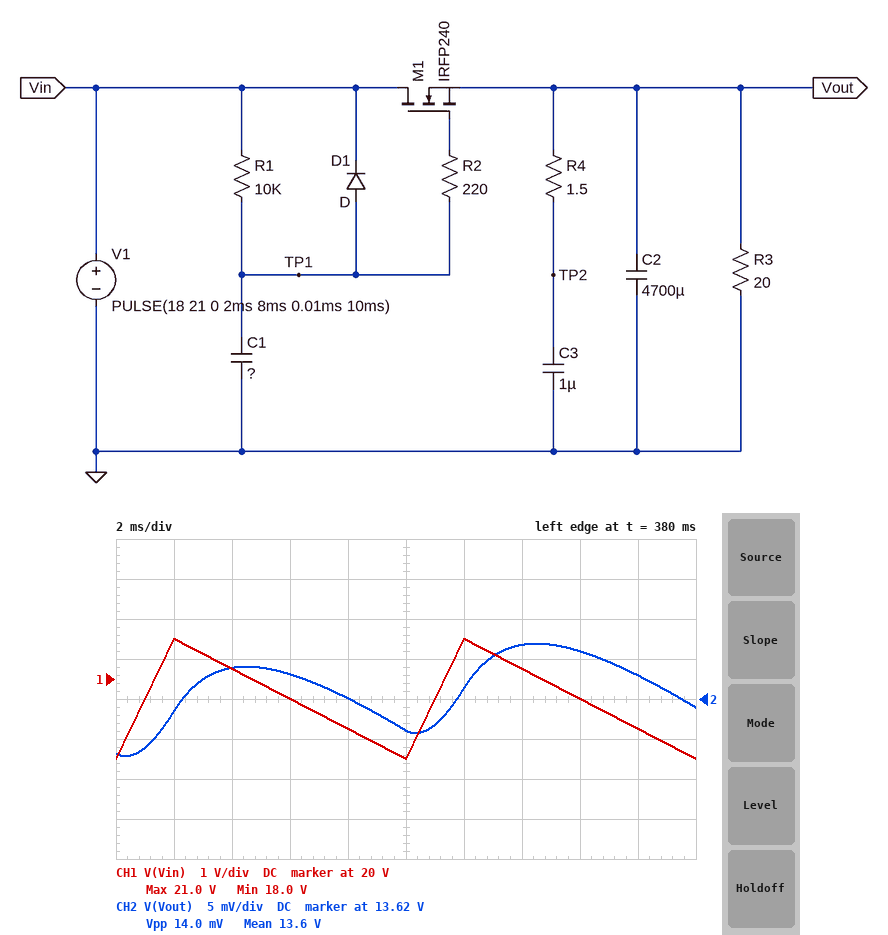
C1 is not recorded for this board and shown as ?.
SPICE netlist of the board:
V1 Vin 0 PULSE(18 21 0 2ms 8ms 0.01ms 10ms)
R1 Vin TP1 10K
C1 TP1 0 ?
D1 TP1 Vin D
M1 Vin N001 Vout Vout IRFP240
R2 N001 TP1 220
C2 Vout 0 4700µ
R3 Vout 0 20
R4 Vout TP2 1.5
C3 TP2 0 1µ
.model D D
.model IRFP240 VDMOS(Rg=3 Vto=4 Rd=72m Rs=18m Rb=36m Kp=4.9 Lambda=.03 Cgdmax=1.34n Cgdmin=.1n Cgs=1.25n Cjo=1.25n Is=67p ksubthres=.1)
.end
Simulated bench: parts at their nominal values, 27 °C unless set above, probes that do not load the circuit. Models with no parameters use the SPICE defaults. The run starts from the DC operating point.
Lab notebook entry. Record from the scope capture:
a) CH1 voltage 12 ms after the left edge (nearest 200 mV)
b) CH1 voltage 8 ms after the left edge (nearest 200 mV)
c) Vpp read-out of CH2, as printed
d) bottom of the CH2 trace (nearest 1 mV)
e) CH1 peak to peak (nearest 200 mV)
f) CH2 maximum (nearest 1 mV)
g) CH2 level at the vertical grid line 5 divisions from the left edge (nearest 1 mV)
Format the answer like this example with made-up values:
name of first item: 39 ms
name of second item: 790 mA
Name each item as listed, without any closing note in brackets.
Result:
CH1 voltage 12 ms after the left edge: 21.0 V
CH1 voltage 8 ms after the left edge: 18.8 V
Vpp read-out of CH2, as printed: 14.0 mV
bottom of the CH2 trace: 13.613 V
CH1 peak to peak: 3.0 V
CH2 maximum: 13.627 V
CH2 level at the vertical grid line 5 divisions from the left edge: 13.616 V
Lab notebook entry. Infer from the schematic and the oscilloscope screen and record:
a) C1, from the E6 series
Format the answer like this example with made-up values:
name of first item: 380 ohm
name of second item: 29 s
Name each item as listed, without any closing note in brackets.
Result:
C1, from the E6 series: 470 µF
